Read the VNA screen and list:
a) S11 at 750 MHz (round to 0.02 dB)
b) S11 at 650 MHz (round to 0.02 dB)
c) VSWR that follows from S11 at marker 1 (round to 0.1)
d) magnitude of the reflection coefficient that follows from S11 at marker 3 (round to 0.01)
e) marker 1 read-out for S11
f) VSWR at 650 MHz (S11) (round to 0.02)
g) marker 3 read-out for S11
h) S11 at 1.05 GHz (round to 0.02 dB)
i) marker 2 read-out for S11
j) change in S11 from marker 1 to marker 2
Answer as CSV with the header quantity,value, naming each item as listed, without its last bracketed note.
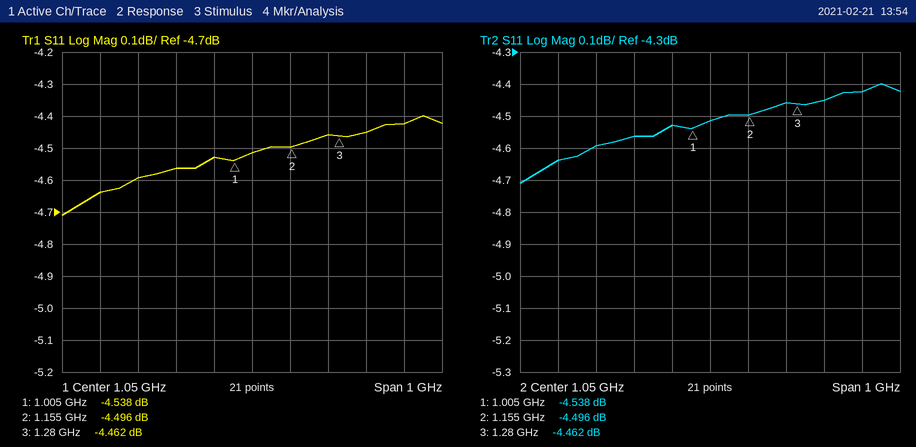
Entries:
quantity,value
S11 at 750 MHz,-4.60 dB
S11 at 650 MHz,-4.64 dB
VSWR that follows from S11 at marker 1,3.9
magnitude of the reflection coefficient that follows from S11 at marker 3,0.60
marker 1 read-out for S11,-4.538 dB
VSWR at 650 MHz (S11),3.84
marker 3 read-out for S11,-4.462 dB
S11 at 1.05 GHz,-4.52 dB
marker 2 read-out for S11,-4.496 dB
change in S11 from marker 1 to marker 2,0.042 dB
